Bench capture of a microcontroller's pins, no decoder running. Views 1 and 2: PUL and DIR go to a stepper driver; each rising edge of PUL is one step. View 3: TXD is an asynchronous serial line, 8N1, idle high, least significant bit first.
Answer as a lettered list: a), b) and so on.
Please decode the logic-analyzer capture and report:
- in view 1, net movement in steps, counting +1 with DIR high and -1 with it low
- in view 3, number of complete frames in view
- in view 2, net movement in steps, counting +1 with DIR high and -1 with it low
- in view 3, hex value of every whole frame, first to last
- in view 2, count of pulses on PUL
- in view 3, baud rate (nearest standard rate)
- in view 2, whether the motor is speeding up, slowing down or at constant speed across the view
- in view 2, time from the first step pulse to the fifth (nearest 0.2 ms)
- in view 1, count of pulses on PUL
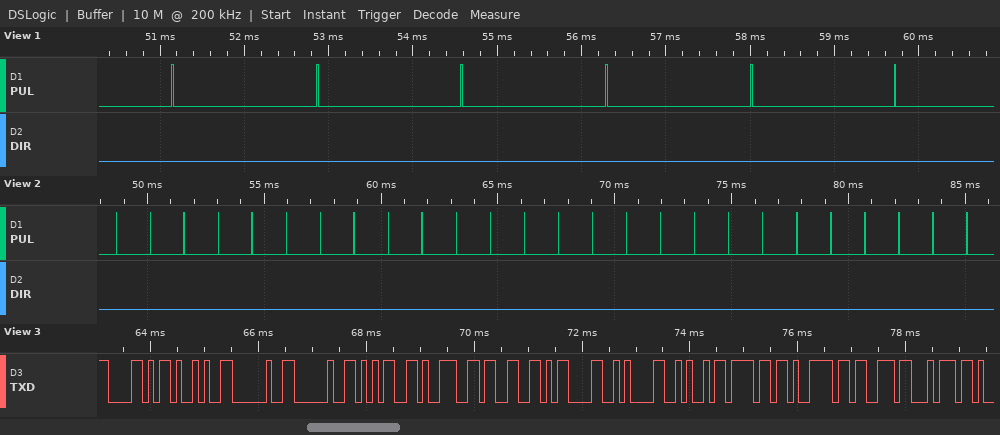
a) -6
b) 14
c) -26
d) 58 29 20 20 35 39 33 0D 0A 4A 6F 79 73 74
e) 26
f) 9600 baud
g) constant speed
h) 5.8 ms
i) 6
